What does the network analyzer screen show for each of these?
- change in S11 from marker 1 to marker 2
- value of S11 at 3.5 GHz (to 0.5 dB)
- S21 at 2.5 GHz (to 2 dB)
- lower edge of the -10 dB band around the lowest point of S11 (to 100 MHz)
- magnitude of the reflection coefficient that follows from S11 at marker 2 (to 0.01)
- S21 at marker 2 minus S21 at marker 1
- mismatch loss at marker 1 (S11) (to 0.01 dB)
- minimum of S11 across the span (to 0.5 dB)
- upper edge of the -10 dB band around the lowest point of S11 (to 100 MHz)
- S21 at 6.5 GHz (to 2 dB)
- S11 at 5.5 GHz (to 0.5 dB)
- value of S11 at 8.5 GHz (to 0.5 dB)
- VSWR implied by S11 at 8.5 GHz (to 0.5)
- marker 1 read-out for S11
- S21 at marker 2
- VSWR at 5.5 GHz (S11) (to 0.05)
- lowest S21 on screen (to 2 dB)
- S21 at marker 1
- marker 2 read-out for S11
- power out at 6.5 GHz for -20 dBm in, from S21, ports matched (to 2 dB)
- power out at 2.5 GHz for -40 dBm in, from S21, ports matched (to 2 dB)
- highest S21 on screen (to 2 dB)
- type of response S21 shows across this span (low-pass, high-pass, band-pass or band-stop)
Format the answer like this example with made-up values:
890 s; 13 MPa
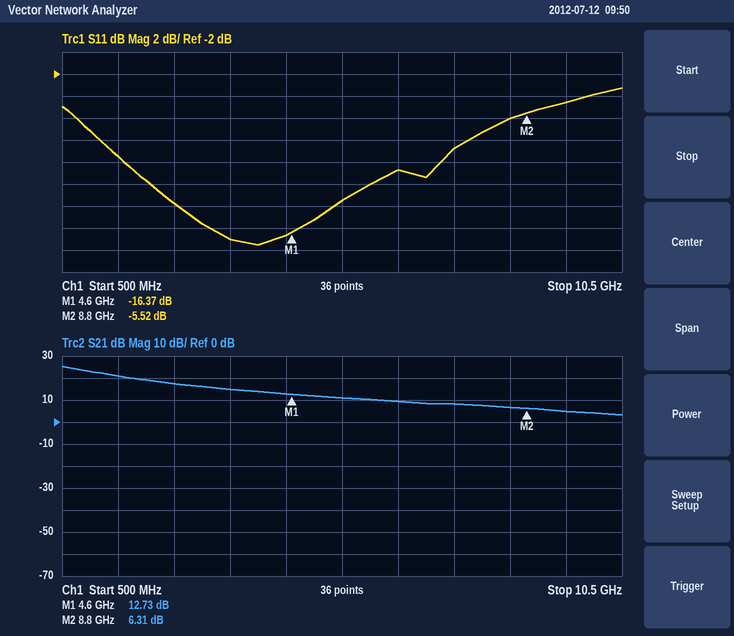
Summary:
10.85 dB; -17.0 dB; 18 dB; 1.6 GHz; 0.53; -6.42 dB; 0.10 dB; -17.5 dB; 7.3 GHz; 10 dB; -13.5 dB; -6.0 dB; 3.0; -16.37 dB; 6.31 dB; 1.55; 4 dB; 12.73 dB; -5.52 dB; -10 dBm; -22 dBm; 26 dB; low-pass
